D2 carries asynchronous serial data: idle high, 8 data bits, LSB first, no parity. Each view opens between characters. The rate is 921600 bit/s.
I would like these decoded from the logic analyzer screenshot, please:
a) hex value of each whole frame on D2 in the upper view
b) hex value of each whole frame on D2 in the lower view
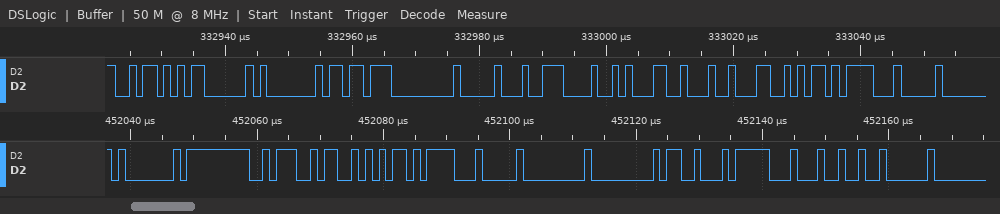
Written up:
5A, 03, 01, DB, 00, 10, 0E, 8A, 22, 4C, EB, 04
01, FF, 3A, 53, EB, 04, 00, 00, 13, 1F, 24, 02
